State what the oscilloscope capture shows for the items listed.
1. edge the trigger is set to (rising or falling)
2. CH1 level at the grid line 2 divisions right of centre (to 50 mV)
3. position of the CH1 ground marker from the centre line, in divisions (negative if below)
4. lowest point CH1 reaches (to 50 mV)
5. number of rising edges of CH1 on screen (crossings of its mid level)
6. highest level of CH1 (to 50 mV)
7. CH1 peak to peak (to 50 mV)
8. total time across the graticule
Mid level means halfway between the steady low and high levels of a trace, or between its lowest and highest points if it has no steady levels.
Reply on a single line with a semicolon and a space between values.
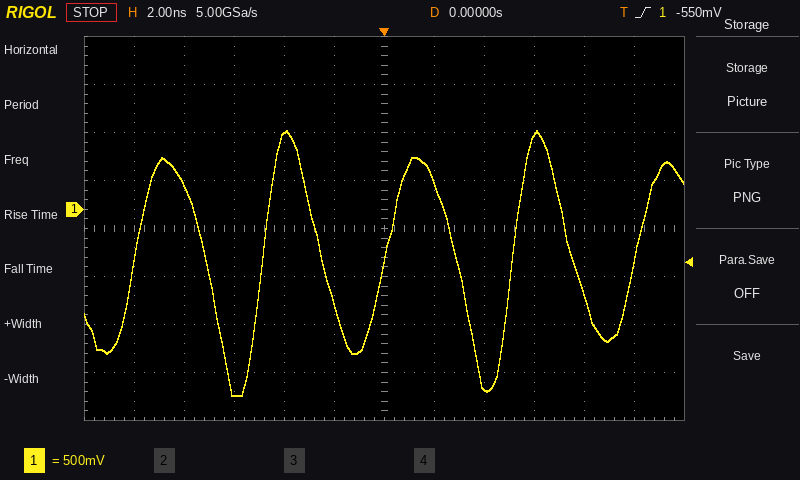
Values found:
rising; -1.85 V; +0.4 div; -1.95 V; 5; 800 mV; 2.75 V; 24 ns
